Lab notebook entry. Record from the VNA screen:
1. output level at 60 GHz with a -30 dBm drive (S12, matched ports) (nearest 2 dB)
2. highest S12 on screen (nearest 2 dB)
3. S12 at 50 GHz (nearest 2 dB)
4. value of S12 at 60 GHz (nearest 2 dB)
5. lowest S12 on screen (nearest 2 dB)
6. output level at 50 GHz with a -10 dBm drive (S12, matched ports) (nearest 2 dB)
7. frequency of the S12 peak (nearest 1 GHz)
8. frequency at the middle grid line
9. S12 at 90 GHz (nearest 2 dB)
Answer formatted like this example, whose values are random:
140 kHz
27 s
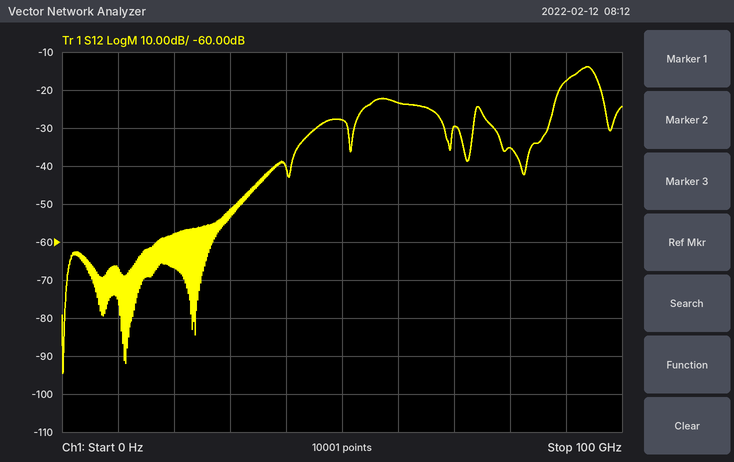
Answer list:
-54 dBm
-14 dB
-28 dB
-24 dB
-94 dB
-38 dBm
94 GHz
50 GHz
-18 dB
